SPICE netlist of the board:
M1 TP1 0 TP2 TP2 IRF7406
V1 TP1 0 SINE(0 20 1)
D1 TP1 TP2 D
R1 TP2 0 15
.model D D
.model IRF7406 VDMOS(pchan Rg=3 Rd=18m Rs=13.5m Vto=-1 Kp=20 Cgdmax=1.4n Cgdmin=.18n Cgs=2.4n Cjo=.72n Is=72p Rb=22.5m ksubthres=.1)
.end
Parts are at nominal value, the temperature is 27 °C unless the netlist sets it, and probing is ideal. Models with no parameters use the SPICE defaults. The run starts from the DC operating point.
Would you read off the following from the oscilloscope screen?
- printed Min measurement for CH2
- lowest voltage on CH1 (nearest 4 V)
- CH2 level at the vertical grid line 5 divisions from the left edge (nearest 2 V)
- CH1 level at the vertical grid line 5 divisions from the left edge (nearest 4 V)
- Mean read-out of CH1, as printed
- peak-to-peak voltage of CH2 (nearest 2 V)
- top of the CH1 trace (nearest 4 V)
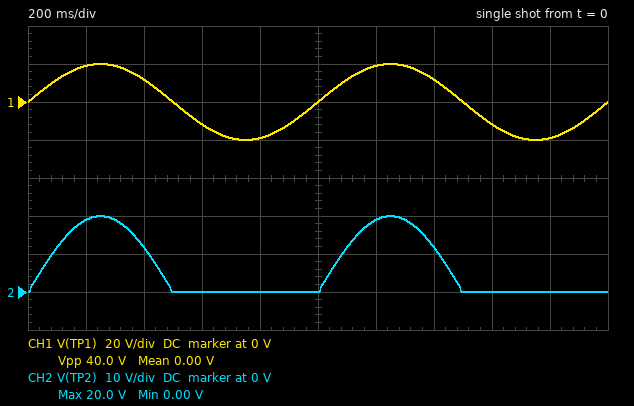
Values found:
0.00 V
-20 V
0 V
0 V
0.00 V
20 V
20 V
